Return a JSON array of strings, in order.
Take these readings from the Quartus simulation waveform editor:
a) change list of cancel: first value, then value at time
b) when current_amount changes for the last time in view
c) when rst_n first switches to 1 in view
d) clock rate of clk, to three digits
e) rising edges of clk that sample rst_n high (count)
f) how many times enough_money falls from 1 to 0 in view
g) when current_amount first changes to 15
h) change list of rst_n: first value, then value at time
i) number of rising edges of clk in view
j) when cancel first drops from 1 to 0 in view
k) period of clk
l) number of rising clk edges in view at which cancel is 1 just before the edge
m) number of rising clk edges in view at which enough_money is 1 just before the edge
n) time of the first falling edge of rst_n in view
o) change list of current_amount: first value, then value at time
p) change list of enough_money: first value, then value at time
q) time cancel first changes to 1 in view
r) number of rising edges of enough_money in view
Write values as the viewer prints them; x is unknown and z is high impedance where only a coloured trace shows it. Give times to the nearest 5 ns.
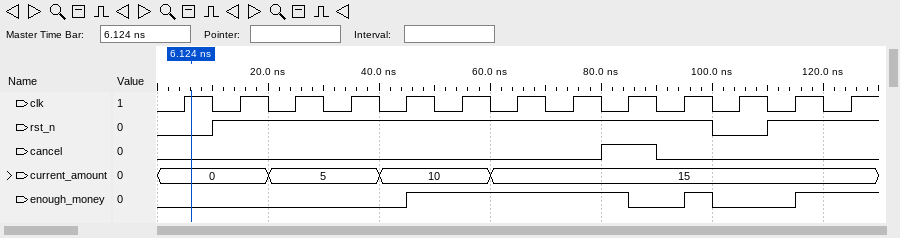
["0, 1 at 80 ns, 0 at 90 ns", "60 ns", "10 ns", "100 MHz", "11", "2", "60 ns", "0, 1 at 10 ns, 0 at 100 ns, 1 at 110 ns", "13", "90 ns", "10 ns", "1", "5", "100 ns", "0, 5 at 20 ns, 10 at 40 ns, 15 at 60 ns", "0, 1 at 45 ns, 0 at 85 ns, 1 at 95 ns, 0 at 100 ns, 1 at 115 ns", "80 ns", "3"]
